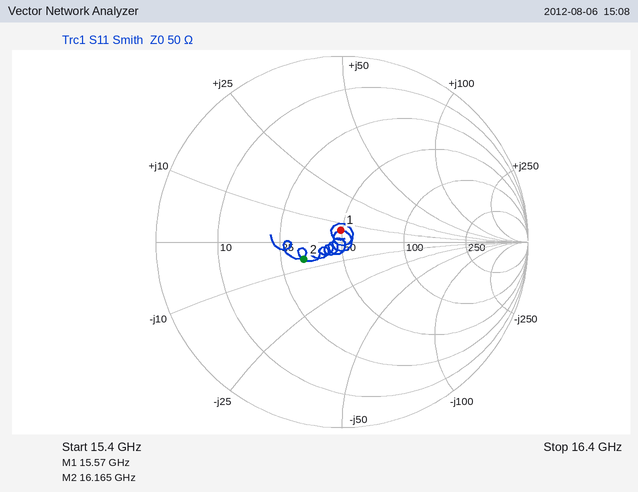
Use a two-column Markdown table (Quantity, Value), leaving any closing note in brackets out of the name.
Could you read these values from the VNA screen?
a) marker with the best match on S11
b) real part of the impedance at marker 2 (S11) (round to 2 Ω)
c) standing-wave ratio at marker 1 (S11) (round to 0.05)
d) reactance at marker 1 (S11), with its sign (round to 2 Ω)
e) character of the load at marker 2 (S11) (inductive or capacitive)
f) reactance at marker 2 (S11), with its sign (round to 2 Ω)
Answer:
| Quantity | Value |
|---|---|
| marker with the best match on S11 | marker 1 |
| real part of the impedance at marker 2 (S11) | 32 Ω |
| standing-wave ratio at marker 1 (S11) | 1.15 |
| reactance at marker 1 (S11), with its sign | +6 Ω |
| character of the load at marker 2 (S11) | capacitive |
| reactance at marker 2 (S11), with its sign | -6 Ω |
